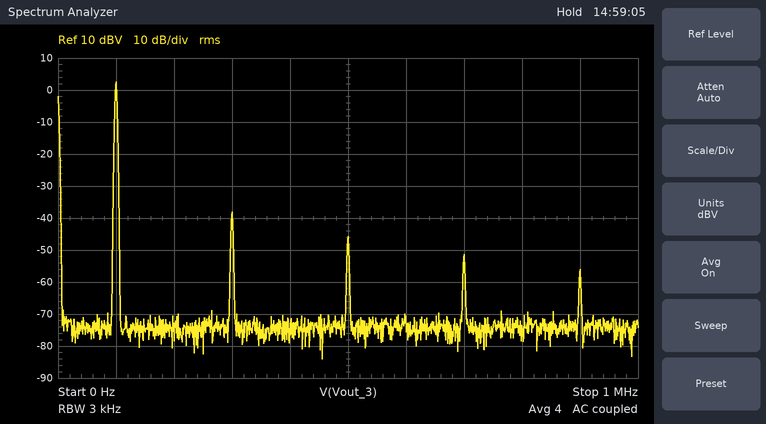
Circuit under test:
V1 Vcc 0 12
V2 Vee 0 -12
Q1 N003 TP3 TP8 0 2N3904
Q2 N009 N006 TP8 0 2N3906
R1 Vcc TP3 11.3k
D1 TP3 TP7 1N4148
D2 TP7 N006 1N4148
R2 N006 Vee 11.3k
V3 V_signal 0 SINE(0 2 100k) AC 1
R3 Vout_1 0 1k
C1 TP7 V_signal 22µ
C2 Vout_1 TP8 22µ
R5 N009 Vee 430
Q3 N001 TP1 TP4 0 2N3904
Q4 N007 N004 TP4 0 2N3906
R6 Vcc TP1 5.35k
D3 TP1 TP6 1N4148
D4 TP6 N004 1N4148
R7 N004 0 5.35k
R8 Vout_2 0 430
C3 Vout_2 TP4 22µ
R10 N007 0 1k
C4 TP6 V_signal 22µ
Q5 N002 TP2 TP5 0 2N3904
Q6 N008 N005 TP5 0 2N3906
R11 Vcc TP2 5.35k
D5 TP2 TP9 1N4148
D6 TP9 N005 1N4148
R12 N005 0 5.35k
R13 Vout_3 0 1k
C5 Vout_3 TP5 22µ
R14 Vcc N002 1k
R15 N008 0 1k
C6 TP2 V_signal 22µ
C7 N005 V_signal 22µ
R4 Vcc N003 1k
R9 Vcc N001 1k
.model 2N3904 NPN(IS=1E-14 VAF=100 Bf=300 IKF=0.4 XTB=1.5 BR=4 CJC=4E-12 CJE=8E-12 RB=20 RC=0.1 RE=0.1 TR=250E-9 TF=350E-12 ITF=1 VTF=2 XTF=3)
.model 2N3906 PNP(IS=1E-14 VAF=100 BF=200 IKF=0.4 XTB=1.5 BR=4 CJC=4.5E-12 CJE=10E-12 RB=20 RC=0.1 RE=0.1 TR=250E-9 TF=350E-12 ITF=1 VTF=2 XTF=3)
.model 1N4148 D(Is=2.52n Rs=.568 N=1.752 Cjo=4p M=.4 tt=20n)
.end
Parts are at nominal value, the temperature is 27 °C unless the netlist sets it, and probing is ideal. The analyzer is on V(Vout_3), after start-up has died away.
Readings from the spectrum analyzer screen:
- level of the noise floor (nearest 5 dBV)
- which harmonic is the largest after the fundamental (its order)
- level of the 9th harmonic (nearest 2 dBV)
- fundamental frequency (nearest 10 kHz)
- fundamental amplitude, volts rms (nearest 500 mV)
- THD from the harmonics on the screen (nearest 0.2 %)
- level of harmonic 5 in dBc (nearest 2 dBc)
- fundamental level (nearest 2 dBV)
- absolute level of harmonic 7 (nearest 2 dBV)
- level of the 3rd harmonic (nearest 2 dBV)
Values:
-75 dBV
3
-56 dBV
100 kHz
1.5 V
1.0 %
-48 dBc
2 dBV
-52 dBV
-38 dBV
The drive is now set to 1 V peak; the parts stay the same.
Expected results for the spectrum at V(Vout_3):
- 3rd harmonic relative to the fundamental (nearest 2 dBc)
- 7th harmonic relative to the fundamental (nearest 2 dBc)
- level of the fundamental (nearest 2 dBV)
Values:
-38 dBc
-56 dBc
-4 dBV
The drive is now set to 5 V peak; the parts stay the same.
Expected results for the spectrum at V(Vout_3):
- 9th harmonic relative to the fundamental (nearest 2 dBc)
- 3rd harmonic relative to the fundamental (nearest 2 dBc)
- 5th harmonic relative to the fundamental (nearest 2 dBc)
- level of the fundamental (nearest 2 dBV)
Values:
-54 dBc
-54 dBc
-56 dBc
10 dBV
